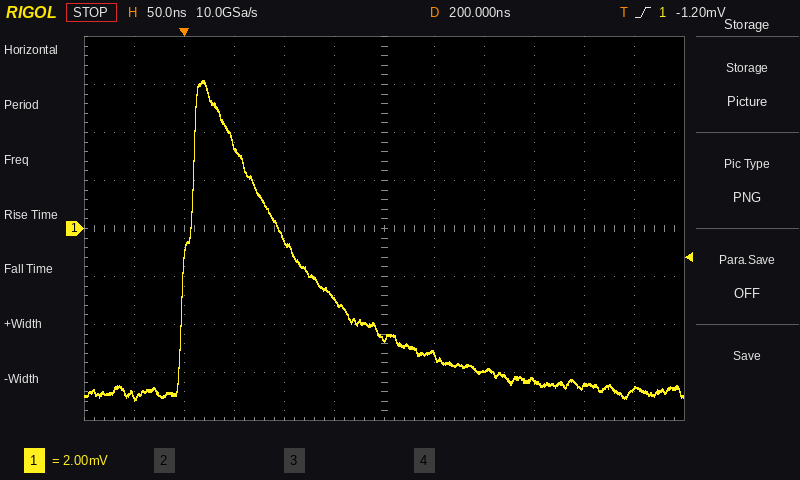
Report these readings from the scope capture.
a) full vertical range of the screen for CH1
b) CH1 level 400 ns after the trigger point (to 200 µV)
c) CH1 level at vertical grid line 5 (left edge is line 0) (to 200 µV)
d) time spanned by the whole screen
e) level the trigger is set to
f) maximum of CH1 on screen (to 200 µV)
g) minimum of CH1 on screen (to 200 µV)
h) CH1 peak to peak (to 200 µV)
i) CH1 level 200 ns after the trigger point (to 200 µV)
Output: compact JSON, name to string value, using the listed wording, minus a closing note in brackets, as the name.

{"full vertical range of the screen for CH1": "16 mV", "CH1 level 400 ns after the trigger point": "-6.6 mV", "CH1 level at vertical grid line 5 (left edge is line 0)": "-3.0 mV", "time spanned by the whole screen": "600 ns", "level the trigger is set to": "-1.20 mV", "maximum of CH1 on screen": "6.2 mV", "minimum of CH1 on screen": "-7.2 mV", "CH1 peak to peak": "13.4 mV", "CH1 level 200 ns after the trigger point": "-4.6 mV"}
